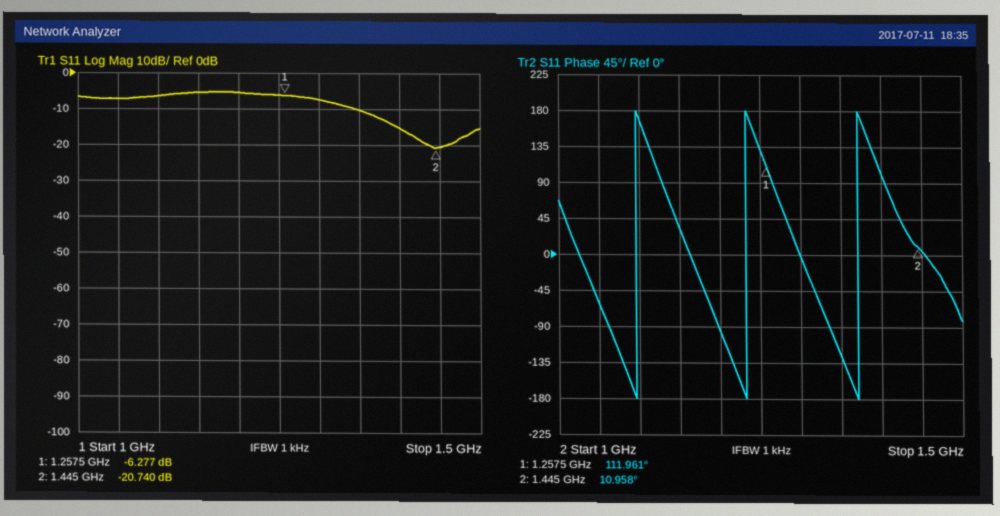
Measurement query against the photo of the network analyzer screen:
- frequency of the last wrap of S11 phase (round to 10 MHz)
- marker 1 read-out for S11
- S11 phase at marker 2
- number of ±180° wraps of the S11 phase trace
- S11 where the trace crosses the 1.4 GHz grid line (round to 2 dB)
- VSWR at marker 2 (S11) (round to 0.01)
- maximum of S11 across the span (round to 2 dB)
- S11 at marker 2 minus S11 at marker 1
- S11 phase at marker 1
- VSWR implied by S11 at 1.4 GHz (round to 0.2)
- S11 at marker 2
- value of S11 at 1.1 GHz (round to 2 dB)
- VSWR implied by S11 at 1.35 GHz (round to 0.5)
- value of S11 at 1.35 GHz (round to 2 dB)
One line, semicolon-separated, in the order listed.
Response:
1.37 GHz; -6.277 dB; 10.958°; 3; -16 dB; 1.20; -6 dB; -14.463 dB; 111.961°; 1.4; -20.740 dB; -6 dB; 2.0; -10 dB
